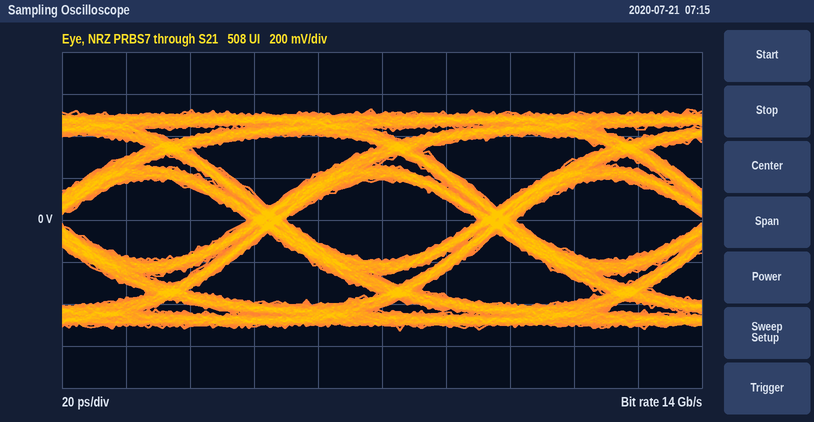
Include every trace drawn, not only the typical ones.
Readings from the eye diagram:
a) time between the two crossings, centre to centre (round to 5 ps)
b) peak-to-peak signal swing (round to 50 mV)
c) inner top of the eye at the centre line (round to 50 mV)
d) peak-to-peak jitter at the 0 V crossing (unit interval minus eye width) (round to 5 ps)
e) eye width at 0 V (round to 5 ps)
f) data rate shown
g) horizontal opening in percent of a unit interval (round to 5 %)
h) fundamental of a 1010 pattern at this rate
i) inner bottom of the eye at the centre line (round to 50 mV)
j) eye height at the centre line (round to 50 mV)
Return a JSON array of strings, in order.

["70 ps", "1.05 V", "200 mV", "10 ps", "60 ps", "14 Gb/s", "85 %", "7 GHz", "-200 mV", "400 mV"]
